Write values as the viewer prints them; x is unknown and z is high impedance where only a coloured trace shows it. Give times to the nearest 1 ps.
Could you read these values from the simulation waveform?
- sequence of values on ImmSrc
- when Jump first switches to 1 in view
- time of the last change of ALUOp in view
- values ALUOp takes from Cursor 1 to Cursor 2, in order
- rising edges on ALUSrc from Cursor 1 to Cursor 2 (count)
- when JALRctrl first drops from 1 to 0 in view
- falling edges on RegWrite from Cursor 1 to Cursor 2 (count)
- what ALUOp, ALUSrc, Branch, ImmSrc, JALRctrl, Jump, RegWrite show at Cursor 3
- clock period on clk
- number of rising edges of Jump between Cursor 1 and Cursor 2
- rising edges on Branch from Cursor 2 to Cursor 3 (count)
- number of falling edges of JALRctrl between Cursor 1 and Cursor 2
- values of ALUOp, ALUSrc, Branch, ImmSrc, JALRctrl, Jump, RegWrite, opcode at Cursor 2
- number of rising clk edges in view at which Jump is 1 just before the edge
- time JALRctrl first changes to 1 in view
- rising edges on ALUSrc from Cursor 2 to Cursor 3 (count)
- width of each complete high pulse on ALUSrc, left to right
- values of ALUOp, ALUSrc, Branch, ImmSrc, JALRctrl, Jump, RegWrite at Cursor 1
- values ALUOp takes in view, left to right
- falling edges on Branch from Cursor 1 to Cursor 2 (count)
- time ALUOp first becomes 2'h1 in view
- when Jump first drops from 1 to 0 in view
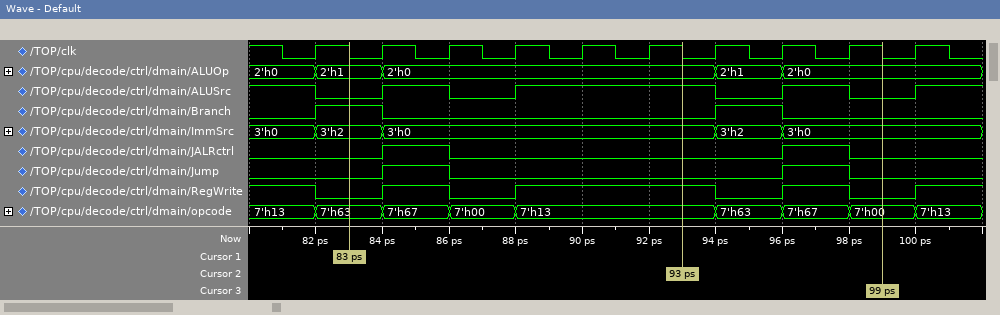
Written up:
3'h0, 3'h2, 3'h0, 3'h2, 3'h0
84 ps
96 ps
2'h1, 2'h0
2
86 ps
1
ALUOp=2'h0, ALUSrc=0, Branch=0, ImmSrc=3'h0, JALRctrl=0, Jump=0, RegWrite=0
2 ps
1
1
1
ALUOp=2'h0, ALUSrc=1, Branch=0, ImmSrc=3'h0, JALRctrl=0, Jump=0, RegWrite=1, opcode=7'h13
2
84 ps
1
2 ps, 6 ps, 2 ps
ALUOp=2'h1, ALUSrc=0, Branch=1, ImmSrc=3'h2, JALRctrl=0, Jump=0, RegWrite=0
2'h0, 2'h1, 2'h0, 2'h1, 2'h0
1
82 ps
86 ps
